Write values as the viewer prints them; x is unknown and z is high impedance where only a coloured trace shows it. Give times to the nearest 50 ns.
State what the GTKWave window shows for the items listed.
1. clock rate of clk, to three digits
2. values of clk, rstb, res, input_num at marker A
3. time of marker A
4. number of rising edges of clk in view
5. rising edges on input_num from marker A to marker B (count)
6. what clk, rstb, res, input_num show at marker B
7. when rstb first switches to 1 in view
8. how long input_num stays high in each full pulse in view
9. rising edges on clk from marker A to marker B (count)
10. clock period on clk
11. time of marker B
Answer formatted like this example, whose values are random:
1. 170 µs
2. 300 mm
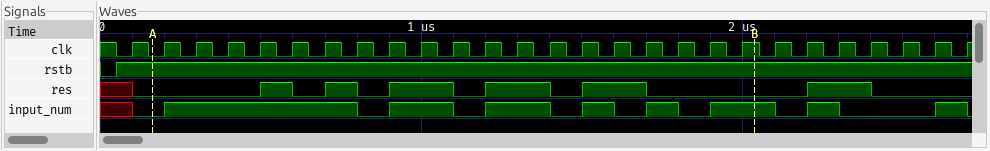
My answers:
1. 10.0 MHz
2. clk=0, rstb=1, res=0, input_num=0
3. 150 ns
4. 27
5. 6
6. clk=1, rstb=1, res=0, input_num=1
7. 50 ns
8. 600 ns, 200 ns, 200 ns, 100 ns, 100 ns, 200 ns, 100 ns, 100 ns
9. 19
10. 100 ns
11. 2050 ns
